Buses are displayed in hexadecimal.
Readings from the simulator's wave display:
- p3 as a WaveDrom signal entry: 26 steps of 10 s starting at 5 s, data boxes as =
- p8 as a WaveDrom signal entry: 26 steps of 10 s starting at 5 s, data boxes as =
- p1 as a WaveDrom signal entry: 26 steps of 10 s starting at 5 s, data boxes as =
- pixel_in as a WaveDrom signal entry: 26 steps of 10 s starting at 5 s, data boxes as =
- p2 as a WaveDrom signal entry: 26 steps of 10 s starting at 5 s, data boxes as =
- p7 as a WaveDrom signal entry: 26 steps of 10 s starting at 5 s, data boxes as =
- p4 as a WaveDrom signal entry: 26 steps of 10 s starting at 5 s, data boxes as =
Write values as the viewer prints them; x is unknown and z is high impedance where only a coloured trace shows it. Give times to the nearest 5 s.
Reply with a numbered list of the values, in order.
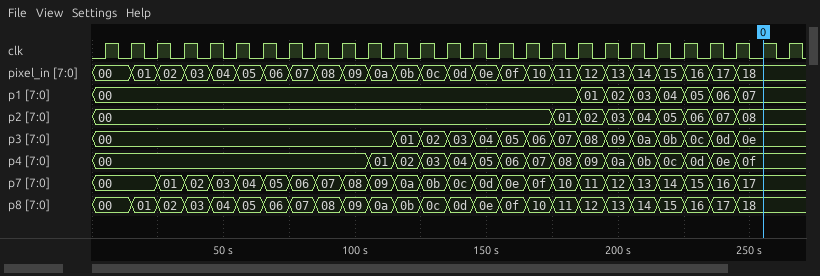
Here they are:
1. {name: 'p3', wave: '=..........==============.', data: '00 01 02 03 04 05 06 07 08 09 0a 0b 0c 0d 0e'}
2. {name: 'p8', wave: '=========================.', data: '00 01 02 03 04 05 06 07 08 09 0a 0b 0c 0d 0e 0f 10 11 12 13 14 15 16 17 18'}
3. {name: 'p1', wave: '=.................=======.', data: '00 01 02 03 04 05 06 07'}
4. {name: 'pixel_in', wave: '=========================.', data: '00 01 02 03 04 05 06 07 08 09 0a 0b 0c 0d 0e 0f 10 11 12 13 14 15 16 17 18'}
5. {name: 'p2', wave: '=................========.', data: '00 01 02 03 04 05 06 07 08'}
6. {name: 'p7', wave: '=.=======================.', data: '00 01 02 03 04 05 06 07 08 09 0a 0b 0c 0d 0e 0f 10 11 12 13 14 15 16 17'}
7. {name: 'p4', wave: '=.........===============.', data: '00 01 02 03 04 05 06 07 08 09 0a 0b 0c 0d 0e 0f'}
